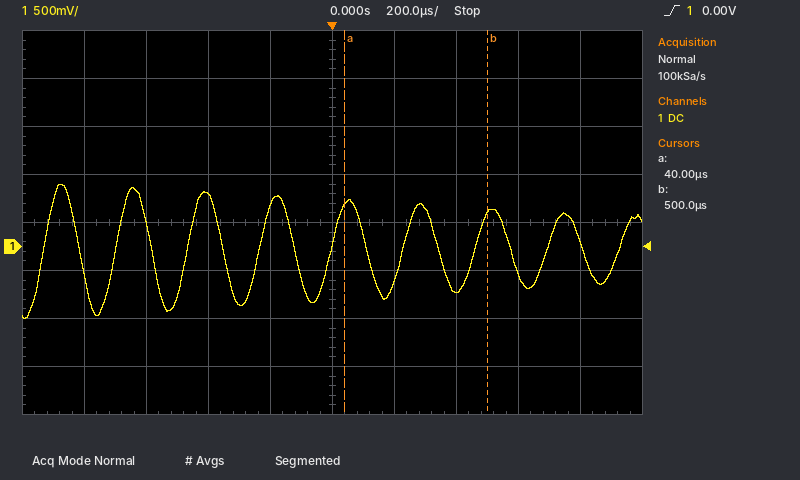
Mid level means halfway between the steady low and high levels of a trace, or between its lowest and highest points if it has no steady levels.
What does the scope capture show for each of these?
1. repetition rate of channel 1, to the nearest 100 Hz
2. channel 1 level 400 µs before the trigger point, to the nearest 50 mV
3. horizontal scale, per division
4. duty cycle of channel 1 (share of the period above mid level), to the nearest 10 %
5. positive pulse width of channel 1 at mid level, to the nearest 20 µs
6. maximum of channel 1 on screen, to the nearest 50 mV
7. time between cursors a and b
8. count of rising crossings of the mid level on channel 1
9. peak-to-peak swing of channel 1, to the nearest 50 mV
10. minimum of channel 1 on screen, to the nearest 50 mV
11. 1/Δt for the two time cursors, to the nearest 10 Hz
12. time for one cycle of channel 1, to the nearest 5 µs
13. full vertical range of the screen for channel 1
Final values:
4.3 kHz
550 mV
200 µs
50 %
120 µs
650 mV
460 µs
9
1.40 V
-750 mV
2.17 kHz
230 µs
4 V
